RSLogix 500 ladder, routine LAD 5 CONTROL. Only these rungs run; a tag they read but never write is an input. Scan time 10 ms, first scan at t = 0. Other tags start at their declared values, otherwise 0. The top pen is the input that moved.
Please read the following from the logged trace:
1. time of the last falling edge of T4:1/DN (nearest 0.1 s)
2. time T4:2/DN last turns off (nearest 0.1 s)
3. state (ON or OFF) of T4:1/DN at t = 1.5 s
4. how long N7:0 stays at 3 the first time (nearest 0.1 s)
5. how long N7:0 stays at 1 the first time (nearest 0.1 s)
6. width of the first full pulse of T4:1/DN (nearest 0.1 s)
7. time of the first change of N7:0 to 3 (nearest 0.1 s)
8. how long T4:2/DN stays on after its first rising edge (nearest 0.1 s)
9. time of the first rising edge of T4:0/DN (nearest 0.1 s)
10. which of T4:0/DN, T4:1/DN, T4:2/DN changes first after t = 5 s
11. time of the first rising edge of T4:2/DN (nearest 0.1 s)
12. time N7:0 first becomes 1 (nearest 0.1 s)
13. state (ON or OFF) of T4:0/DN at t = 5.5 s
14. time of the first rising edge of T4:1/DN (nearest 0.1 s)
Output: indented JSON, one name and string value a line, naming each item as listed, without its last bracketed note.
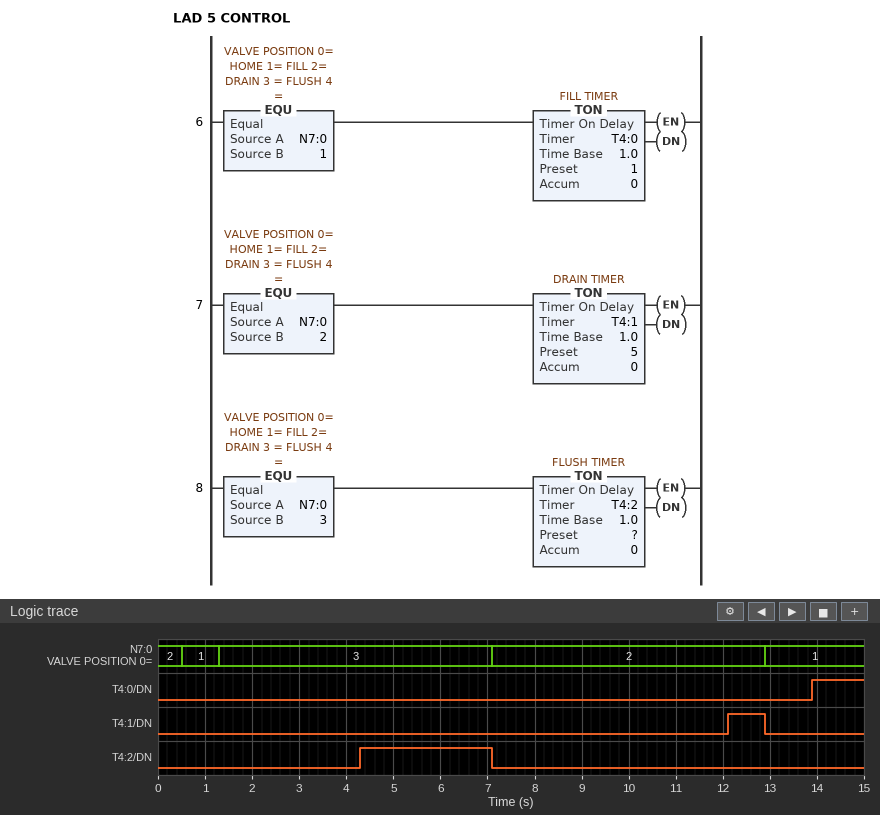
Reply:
{
  "time of the last falling edge of T4:1/DN": "12.9 s",
  "time T4:2/DN last turns off": "7.1 s",
  "state (ON or OFF) of T4:1/DN at t = 1.5 s": "OFF",
  "how long N7:0 stays at 3 the first time": "5.8 s",
  "how long N7:0 stays at 1 the first time": "0.8 s",
  "width of the first full pulse of T4:1/DN": "0.8 s",
  "time of the first change of N7:0 to 3": "1.3 s",
  "how long T4:2/DN stays on after its first rising edge": "2.8 s",
  "time of the first rising edge of T4:0/DN": "13.9 s",
  "which of T4:0/DN, T4:1/DN, T4:2/DN changes first after t = 5 s": "T4:2/DN",
  "time of the first rising edge of T4:2/DN": "4.3 s",
  "time N7:0 first becomes 1": "0.5 s",
  "state (ON or OFF) of T4:0/DN at t = 5.5 s": "OFF",
  "time of the first rising edge of T4:1/DN": "12.1 s"
}
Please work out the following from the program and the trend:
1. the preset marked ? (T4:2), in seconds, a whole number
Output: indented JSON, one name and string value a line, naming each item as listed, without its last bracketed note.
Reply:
{
  "the preset marked ? (T4:2), in seconds, a whole number": "3 s"
}
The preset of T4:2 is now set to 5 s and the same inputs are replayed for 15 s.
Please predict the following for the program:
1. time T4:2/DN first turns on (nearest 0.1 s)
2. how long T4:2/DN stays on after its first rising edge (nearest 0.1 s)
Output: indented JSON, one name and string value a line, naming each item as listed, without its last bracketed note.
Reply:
{
  "time T4:2/DN first turns on": "6.3 s",
  "how long T4:2/DN stays on after its first rising edge": "0.8 s"
}
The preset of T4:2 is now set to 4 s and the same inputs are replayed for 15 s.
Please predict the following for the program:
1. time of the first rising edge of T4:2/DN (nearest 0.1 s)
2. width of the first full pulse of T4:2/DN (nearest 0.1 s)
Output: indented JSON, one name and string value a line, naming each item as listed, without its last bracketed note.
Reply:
{
  "time of the first rising edge of T4:2/DN": "5.3 s",
  "width of the first full pulse of T4:2/DN": "1.8 s"
}
